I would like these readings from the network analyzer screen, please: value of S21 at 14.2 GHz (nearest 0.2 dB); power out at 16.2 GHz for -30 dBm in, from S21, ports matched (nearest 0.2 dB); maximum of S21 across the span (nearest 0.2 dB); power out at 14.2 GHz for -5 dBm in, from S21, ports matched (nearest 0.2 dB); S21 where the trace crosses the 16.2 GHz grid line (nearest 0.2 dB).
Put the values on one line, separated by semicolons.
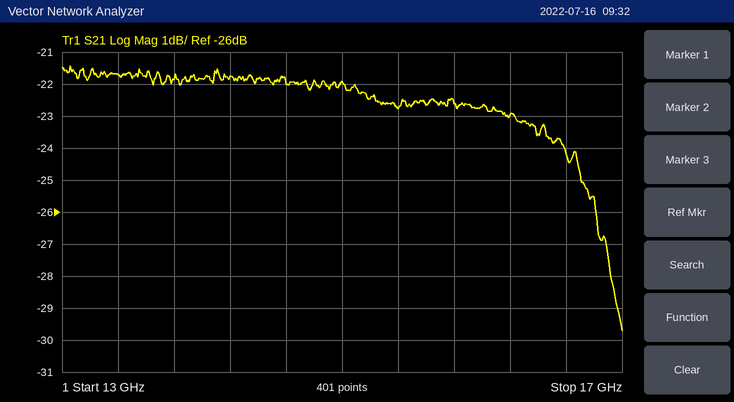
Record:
-21.8 dB; -53.0 dBm; -21.4 dB; -26.8 dBm; -23.0 dB
